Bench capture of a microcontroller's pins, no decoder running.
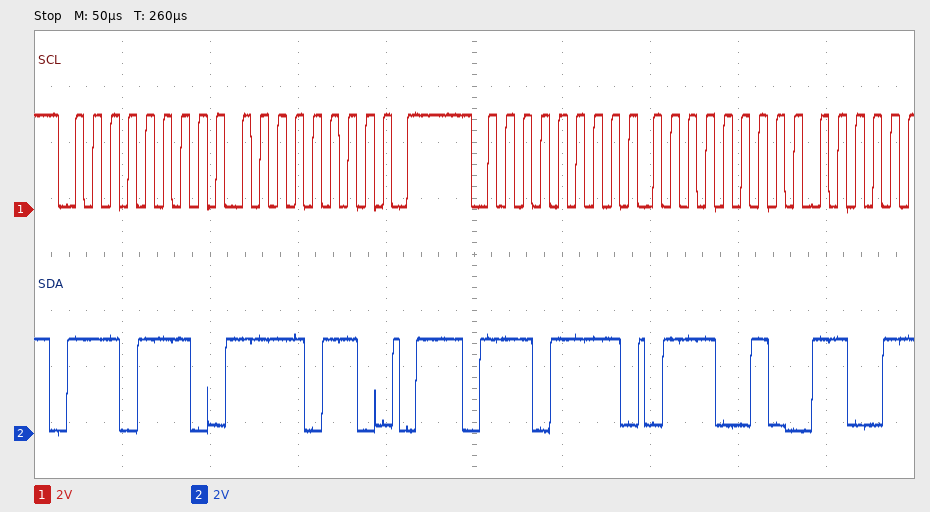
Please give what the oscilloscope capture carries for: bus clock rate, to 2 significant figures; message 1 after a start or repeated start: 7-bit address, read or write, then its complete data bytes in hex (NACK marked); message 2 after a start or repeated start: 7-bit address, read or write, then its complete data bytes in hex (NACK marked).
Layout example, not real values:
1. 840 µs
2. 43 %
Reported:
1. 100 kHz
2. 0x77 write: F6
3. 0x77 read: 72
